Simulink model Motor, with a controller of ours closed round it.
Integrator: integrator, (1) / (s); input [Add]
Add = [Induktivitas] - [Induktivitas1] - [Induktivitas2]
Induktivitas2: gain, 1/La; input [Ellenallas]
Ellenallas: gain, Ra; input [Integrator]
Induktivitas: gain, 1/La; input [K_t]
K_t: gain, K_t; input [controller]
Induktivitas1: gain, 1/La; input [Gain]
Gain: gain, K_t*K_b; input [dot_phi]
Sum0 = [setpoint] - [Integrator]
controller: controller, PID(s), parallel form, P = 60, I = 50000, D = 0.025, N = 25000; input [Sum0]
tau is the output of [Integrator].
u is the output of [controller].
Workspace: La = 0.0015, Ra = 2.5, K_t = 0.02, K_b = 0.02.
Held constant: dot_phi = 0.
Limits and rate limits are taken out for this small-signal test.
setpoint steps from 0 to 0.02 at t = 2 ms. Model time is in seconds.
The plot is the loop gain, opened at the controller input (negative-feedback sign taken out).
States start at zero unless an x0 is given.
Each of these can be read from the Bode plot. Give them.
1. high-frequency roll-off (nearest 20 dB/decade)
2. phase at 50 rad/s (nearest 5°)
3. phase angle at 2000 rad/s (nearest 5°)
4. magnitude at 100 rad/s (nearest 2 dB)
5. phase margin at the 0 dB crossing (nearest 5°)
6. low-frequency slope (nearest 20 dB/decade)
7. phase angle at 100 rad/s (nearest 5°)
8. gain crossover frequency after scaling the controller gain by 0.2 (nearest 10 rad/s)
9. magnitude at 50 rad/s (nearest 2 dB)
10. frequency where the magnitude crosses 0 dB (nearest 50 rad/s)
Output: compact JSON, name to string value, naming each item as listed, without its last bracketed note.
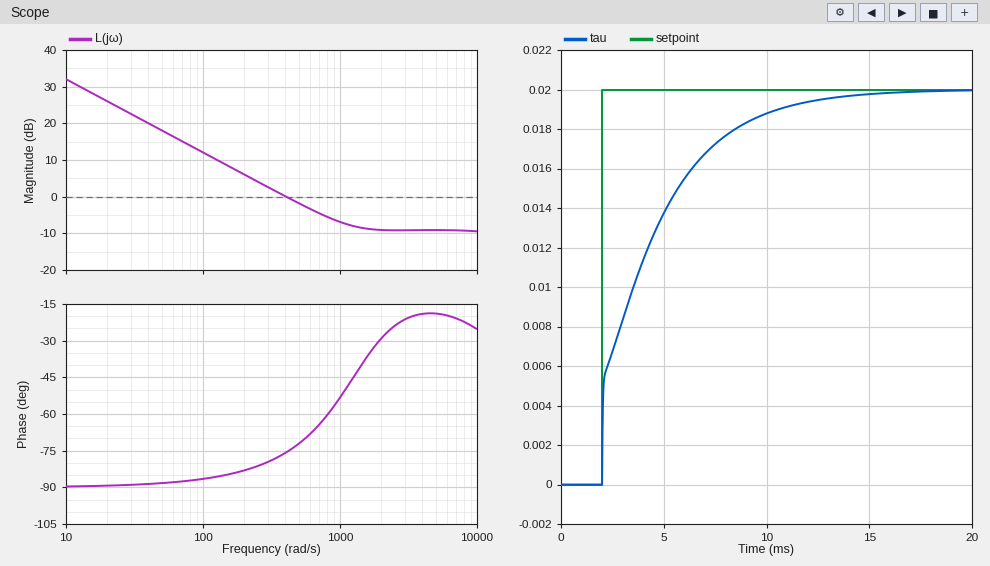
{"high-frequency roll-off": "0 dB/decade", "phase at 50 rad/s": "-90°", "phase angle at 2000 rad/s": "-30°", "magnitude at 100 rad/s": "12 dB", "phase margin at the 0 dB crossing": "105°", "low-frequency slope": "-20 dB/decade", "phase angle at 100 rad/s": "-85°", "gain crossover frequency after scaling the controller gain by 0.2": "80 rad/s", "magnitude at 50 rad/s": "18 dB", "frequency where the magnitude crosses 0 dB": "400 rad/s"}
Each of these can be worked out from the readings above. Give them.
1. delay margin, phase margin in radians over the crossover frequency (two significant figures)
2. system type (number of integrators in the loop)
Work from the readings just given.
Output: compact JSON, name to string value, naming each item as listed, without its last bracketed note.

{"delay margin, phase margin in radians over the crossover frequency": "0.0046 s", "system type": "1"}
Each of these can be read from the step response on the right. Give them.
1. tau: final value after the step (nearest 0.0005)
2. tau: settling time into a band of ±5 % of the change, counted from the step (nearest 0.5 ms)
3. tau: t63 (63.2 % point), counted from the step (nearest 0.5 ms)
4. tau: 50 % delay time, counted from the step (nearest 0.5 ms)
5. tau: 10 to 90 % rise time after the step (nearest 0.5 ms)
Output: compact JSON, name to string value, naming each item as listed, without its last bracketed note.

{"tau: final value after the step": "0.0200", "tau: settling time into a band of ±5 % of the change, counted from the step": "8.5 ms", "tau: t63 (63.2 % point), counted from the step": "2.5 ms", "tau: 50 % delay time, counted from the step": "1.5 ms", "tau: 10 to 90 % rise time after the step": "6.5 ms"}
